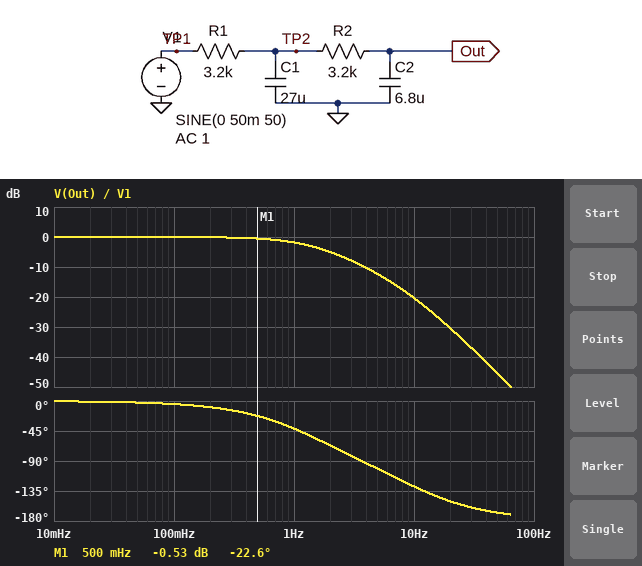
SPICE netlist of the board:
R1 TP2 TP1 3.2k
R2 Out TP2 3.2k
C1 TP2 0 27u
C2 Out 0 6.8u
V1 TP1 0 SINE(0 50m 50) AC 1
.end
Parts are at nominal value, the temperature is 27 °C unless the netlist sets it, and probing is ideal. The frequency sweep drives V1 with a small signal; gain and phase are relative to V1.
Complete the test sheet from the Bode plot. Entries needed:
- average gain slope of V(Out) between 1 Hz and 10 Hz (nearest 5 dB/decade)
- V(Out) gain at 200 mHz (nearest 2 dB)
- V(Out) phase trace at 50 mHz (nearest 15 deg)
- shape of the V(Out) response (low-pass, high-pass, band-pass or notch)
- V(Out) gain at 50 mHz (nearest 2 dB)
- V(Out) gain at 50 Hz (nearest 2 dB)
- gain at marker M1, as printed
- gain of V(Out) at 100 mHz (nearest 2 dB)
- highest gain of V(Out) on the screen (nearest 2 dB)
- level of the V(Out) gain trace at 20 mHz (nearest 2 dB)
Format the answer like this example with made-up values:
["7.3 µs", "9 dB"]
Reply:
["-20 dB/decade", "0 dB", "0 deg", "low-pass", "0 dB", "-46 dB", "-0.53 dB", "0 dB", "0 dB", "0 dB"]
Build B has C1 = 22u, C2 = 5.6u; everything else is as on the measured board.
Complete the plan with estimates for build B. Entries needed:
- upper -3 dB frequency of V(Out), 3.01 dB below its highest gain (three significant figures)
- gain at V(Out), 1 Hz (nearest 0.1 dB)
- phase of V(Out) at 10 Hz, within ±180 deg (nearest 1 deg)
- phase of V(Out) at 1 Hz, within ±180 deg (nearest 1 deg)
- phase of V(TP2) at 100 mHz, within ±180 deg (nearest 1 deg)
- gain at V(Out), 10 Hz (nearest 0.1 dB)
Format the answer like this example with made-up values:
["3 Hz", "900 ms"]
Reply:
["1.68 Hz", "-1.3 dB", "-121 deg", "-35 deg", "-3 deg", "-17.8 dB"]
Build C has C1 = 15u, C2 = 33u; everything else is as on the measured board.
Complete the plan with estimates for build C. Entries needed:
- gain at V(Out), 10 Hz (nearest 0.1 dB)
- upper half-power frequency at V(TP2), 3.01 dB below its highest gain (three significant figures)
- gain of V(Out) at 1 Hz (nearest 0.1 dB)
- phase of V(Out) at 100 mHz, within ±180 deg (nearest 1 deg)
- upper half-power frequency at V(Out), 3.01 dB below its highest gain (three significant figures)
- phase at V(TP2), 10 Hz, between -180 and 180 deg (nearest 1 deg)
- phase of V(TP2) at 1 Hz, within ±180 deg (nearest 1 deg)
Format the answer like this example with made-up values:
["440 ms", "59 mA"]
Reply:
["-28.0 dB", "845 mHz", "-5.2 dB", "-9 deg", "664 mHz", "-58 deg", "-30 deg"]
